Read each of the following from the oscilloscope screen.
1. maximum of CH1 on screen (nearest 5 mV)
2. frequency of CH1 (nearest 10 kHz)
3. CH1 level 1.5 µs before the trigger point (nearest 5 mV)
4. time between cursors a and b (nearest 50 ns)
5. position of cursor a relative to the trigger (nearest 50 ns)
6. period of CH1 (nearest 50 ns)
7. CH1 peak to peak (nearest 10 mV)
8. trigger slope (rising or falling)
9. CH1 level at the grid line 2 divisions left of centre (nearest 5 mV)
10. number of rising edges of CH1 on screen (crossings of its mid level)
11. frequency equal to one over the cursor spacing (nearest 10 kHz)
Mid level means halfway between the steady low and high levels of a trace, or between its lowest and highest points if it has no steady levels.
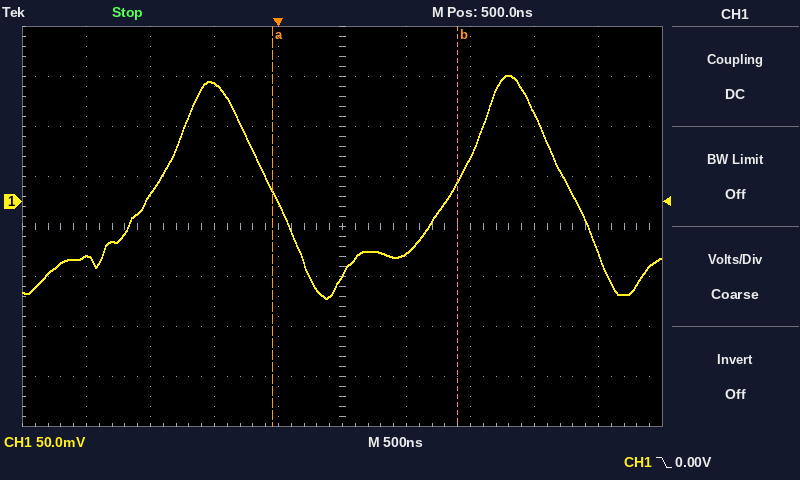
125 mV
430 kHz
-55 mV
1.45 µs
-50 ns
2.35 µs
220 mV
falling
120 mV
2
690 kHz
